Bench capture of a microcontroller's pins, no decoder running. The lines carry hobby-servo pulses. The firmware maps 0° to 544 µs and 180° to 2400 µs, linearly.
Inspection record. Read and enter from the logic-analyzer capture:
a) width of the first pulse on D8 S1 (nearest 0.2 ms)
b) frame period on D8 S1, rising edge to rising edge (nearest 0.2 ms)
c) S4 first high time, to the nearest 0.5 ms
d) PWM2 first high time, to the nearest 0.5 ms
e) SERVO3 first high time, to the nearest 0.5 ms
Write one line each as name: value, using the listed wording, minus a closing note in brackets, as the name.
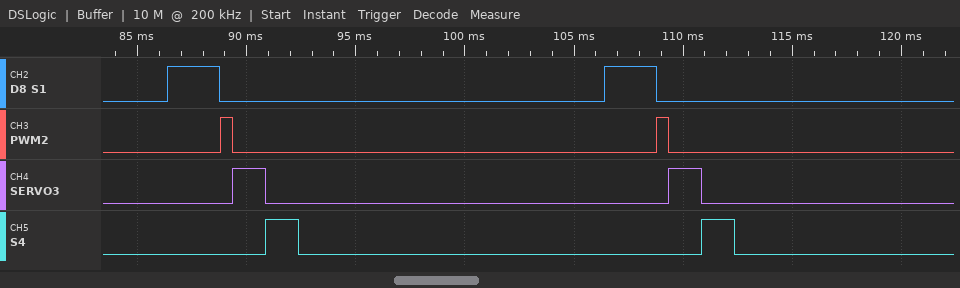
width of the first pulse on D8 S1: 2.4 ms
frame period on D8 S1, rising edge to rising edge: 20.0 ms
S4 first high time, to the nearest 0.5 ms: 1.5 ms
PWM2 first high time, to the nearest 0.5 ms: 0.5 ms
SERVO3 first high time, to the nearest 0.5 ms: 1.5 ms
